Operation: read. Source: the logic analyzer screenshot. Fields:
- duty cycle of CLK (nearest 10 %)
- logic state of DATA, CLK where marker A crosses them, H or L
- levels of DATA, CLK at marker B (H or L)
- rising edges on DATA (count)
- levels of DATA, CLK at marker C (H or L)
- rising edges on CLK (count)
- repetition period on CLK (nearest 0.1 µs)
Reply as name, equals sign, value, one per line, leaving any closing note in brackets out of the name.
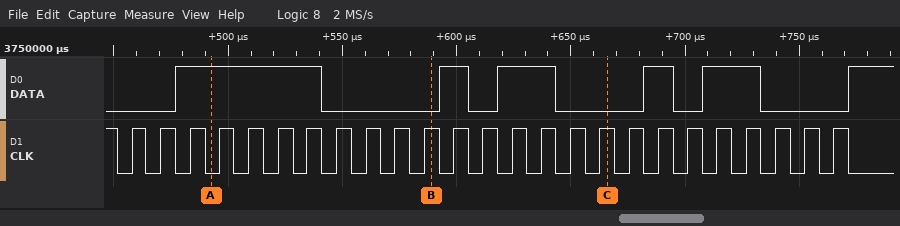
duty cycle of CLK = 50 %
logic state of DATA, CLK where marker A crosses them, H or L = DATA=H, CLK=L
levels of DATA, CLK at marker B = DATA=L, CLK=H
rising edges on DATA = 6
levels of DATA, CLK at marker C = DATA=L, CLK=H
rising edges on CLK = 25
repetition period on CLK = 12.8 µs
